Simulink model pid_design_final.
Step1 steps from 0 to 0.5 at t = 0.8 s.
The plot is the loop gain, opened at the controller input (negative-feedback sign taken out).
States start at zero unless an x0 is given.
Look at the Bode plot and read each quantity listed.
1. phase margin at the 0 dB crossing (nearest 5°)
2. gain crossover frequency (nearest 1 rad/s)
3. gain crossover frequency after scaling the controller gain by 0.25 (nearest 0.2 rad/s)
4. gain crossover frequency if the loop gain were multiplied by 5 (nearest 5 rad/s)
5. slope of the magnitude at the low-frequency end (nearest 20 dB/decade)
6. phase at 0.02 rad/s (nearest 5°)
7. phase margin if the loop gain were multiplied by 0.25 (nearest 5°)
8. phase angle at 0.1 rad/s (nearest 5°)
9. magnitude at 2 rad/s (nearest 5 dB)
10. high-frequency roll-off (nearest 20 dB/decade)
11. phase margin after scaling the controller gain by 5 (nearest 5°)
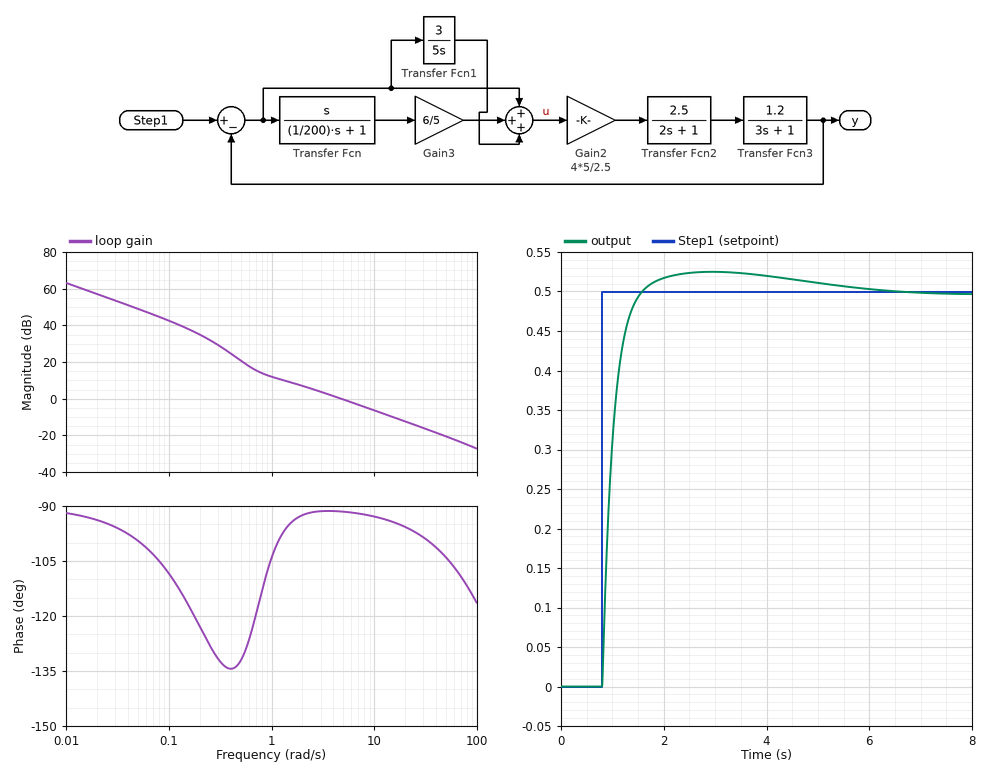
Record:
90°
5 rad/s
1.0 rad/s
25 rad/s
-20 dB/decade
-95°
75°
-110°
5 dB
-20 dB/decade
85°
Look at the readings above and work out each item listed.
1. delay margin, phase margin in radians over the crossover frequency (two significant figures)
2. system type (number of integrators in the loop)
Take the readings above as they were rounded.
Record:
0.31 s
1
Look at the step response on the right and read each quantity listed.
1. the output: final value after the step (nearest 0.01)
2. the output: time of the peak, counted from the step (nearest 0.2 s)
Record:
0.50
2.2 s
